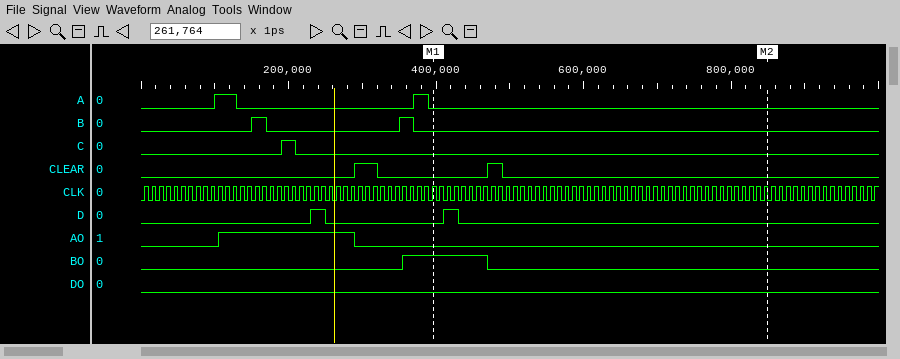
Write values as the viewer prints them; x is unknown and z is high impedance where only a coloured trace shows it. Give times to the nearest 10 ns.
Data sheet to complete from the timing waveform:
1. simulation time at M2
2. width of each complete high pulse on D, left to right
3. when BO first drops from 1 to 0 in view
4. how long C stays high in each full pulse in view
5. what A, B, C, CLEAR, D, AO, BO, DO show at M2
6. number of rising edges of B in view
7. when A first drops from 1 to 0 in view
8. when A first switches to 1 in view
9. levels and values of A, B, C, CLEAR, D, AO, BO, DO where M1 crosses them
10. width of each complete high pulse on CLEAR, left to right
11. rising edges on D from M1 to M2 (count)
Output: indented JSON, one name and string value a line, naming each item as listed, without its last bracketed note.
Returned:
{
  "simulation time at M2": "850 ns",
  "width of each complete high pulse on D, left to right": "20 ns, 20 ns",
  "when BO first drops from 1 to 0 in view": "470 ns",
  "how long C stays high in each full pulse in view": "20 ns",
  "what A, B, C, CLEAR, D, AO, BO, DO show at M2": "A=0, B=0, C=0, CLEAR=0, D=0, AO=0, BO=0, DO=0",
  "number of rising edges of B in view": "2",
  "when A first drops from 1 to 0 in view": "130 ns",
  "when A first switches to 1 in view": "100 ns",
  "levels and values of A, B, C, CLEAR, D, AO, BO, DO where M1 crosses them": "A=0, B=0, C=0, CLEAR=0, D=0, AO=0, BO=1, DO=0",
  "width of each complete high pulse on CLEAR, left to right": "30 ns, 20 ns",
  "rising edges on D from M1 to M2": "1"
}
